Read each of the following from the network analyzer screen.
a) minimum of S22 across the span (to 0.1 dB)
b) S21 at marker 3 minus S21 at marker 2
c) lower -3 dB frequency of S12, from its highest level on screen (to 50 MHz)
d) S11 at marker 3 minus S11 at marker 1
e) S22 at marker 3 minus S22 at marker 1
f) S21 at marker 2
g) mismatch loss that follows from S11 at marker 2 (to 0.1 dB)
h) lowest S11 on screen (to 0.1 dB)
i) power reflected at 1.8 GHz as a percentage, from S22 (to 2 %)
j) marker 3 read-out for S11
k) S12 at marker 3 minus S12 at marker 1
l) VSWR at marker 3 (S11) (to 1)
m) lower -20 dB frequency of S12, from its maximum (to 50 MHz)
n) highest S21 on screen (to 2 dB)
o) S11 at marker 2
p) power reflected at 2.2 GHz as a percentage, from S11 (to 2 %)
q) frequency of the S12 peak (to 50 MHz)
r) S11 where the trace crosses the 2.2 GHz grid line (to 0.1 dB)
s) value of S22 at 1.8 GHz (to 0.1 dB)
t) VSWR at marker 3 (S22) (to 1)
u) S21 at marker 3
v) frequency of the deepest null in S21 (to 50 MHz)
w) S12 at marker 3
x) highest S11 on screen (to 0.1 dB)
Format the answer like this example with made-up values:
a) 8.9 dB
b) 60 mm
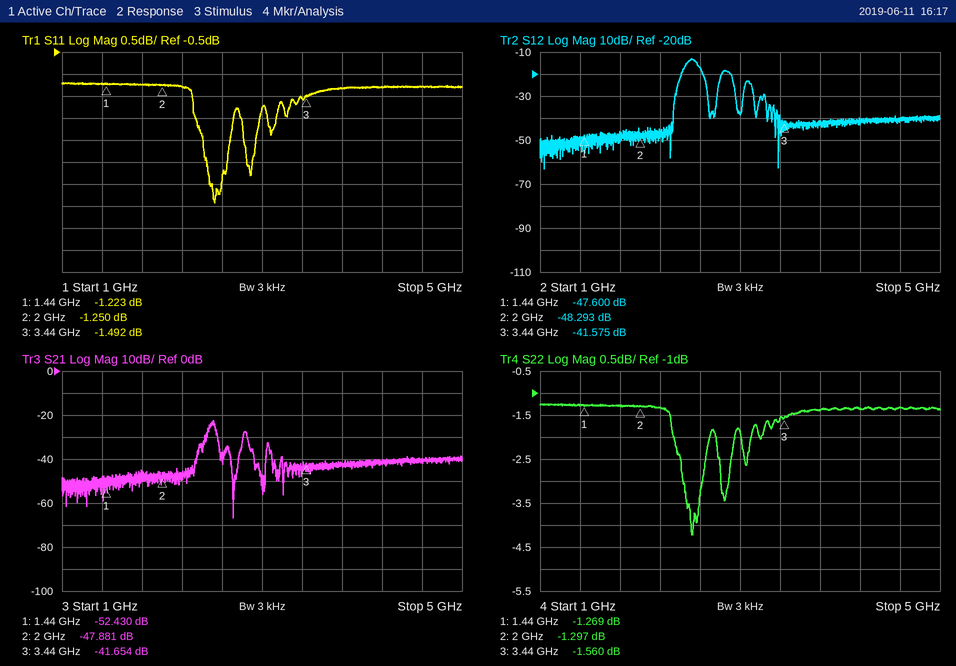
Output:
a) -4.2 dB
b) 6.227 dB
c) 2.45 GHz
d) -0.269 dB
e) -0.291 dB
f) -47.881 dB
g) 6.0 dB
h) -3.9 dB
i) 74 %
j) -1.492 dB
k) 6.025 dB
l) 12
m) 2.35 GHz
n) -22 dB
o) -1.250 dB
p) 74 %
q) 2.50 GHz
r) -1.3 dB
s) -1.3 dB
t) 11
u) -41.654 dB
v) 2.70 GHz
w) -41.575 dB
x) -1.2 dB
